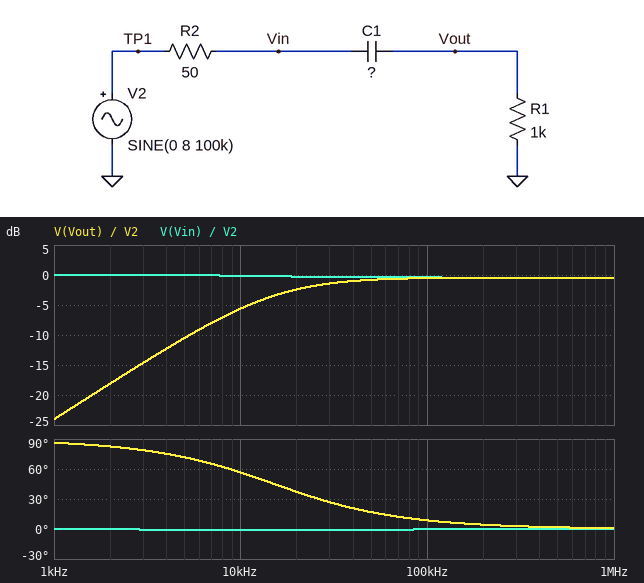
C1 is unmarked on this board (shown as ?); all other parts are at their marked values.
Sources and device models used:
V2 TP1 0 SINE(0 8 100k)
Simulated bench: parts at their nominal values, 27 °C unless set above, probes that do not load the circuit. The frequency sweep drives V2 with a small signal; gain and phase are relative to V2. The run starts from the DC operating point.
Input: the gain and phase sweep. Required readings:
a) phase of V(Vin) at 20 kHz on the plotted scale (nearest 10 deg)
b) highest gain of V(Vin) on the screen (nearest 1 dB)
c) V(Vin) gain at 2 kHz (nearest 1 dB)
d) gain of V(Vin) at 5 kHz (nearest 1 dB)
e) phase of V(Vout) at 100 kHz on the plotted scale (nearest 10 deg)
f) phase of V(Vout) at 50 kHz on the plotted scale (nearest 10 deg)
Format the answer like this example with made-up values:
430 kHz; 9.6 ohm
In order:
0 deg; 0 dB; 0 dB; 0 dB; 10 deg; 20 deg
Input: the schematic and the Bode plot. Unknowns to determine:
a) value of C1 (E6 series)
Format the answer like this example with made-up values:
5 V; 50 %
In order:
10 nF
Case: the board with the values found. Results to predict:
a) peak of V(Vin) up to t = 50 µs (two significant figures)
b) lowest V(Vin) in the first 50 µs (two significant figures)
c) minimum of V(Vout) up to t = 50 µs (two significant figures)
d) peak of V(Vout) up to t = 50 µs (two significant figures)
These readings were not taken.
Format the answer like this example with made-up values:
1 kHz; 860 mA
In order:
7.7 V; -7.6 V; -8.1 V; 7.5 V
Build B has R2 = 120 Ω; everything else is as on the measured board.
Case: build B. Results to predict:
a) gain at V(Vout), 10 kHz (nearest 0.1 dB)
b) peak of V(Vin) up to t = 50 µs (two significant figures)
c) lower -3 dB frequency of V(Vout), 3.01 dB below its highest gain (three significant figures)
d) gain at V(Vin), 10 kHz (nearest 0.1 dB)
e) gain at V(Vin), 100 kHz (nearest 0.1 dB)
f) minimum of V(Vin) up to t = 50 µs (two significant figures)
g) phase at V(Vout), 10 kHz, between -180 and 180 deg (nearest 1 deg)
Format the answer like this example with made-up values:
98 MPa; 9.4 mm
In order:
-5.8 dB; 7.3 V; 14.2 kHz; -0.3 dB; -1.0 dB; -7.2 V; 55 deg
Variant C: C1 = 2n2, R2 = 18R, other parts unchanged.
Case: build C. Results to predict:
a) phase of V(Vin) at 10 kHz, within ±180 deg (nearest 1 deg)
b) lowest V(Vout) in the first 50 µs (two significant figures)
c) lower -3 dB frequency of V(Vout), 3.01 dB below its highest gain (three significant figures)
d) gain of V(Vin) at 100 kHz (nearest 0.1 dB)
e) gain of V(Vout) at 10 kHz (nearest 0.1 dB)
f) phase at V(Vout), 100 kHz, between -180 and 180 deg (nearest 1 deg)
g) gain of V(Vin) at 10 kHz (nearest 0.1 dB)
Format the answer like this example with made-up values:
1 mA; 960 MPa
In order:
0 deg; -6.6 V; 71.1 kHz; -0.1 dB; -17.3 dB; 35 deg; 0 dB
